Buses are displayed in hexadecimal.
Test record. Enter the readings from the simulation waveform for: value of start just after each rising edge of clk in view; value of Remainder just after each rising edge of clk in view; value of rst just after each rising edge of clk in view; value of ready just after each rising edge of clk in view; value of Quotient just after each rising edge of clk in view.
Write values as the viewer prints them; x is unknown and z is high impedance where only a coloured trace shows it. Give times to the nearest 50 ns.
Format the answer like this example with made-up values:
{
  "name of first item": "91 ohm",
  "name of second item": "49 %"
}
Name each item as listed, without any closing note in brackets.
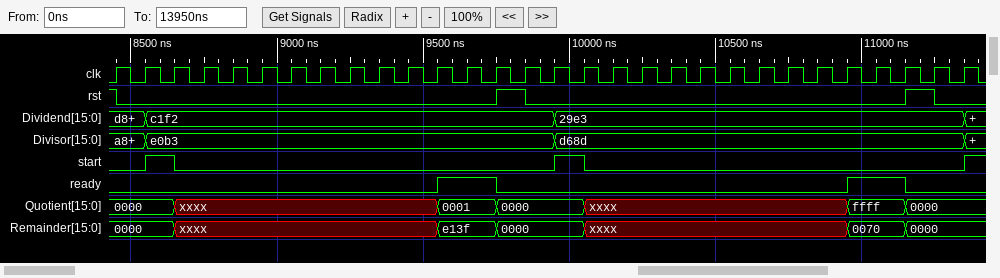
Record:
{
  "value of start just after each rising edge of clk in view": "0 1 0 0 0 0 0 0 0 0 0 0 0 0 0 1 0 0 0 0 0 0 0 0 0 0 0 0 0 1",
  "value of Remainder just after each rising edge of clk in view": "0000, 0000, xxxx, xxxx, xxxx, xxxx, xxxx, xxxx, xxxx, xxxx, xxxx, e13f, e13f, 0000, 0000, 0000, xxxx, xxxx, xxxx, xxxx, xxxx, xxxx, xxxx, xxxx, xxxx, 0070, 0070, 0000, 0000, 0000",
  "value of rst just after each rising edge of clk in view": "0 0 0 0 0 0 0 0 0 0 0 0 0 1 0 0 0 0 0 0 0 0 0 0 0 0 0 1 0 0",
  "value of ready just after each rising edge of clk in view": "0 0 0 0 0 0 0 0 0 0 0 1 1 0 0 0 0 0 0 0 0 0 0 0 0 1 1 0 0 0",
  "value of Quotient just after each rising edge of clk in view": "0000, 0000, xxxx, xxxx, xxxx, xxxx, xxxx, xxxx, xxxx, xxxx, xxxx, 0001, 0001, 0000, 0000, 0000, xxxx, xxxx, xxxx, xxxx, xxxx, xxxx, xxxx, xxxx, xxxx, ffff, ffff, 0000, 0000, 0000"
}
